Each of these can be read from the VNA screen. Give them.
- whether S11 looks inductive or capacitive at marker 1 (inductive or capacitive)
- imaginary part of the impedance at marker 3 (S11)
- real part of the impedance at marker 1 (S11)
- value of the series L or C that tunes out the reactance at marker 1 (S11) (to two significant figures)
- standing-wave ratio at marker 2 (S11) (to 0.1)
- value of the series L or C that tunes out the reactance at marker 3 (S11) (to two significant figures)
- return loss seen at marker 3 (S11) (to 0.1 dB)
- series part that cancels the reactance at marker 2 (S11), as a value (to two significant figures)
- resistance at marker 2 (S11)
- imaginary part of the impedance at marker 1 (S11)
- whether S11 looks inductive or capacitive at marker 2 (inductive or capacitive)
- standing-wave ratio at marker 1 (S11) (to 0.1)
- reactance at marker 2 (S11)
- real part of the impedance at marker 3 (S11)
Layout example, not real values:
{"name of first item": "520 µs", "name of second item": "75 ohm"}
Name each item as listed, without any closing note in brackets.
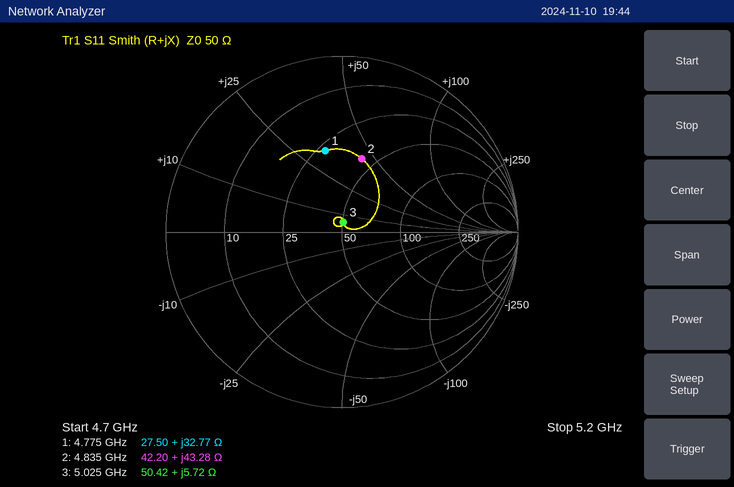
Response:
{"whether S11 looks inductive or capacitive at marker 1": "inductive", "imaginary part of the impedance at marker 3": "+5.72 Ω", "real part of the impedance at marker 1": "27.50 Ω", "value of the series L or C that tunes out the reactance at marker 1 (S11)": "1.0 pF", "standing-wave ratio at marker 2 (S11)": "2.5", "value of the series L or C that tunes out the reactance at marker 3 (S11)": "5.5 pF", "return loss seen at marker 3 (S11)": "24.9 dB", "series part that cancels the reactance at marker 2 (S11), as a value": "760 fF", "resistance at marker 2": "42.20 Ω", "imaginary part of the impedance at marker 1": "+32.77 Ω", "whether S11 looks inductive or capacitive at marker 2": "inductive", "standing-wave ratio at marker 1 (S11)": "2.8", "reactance at marker 2": "+43.28 Ω", "real part of the impedance at marker 3": "50.42 Ω"}
